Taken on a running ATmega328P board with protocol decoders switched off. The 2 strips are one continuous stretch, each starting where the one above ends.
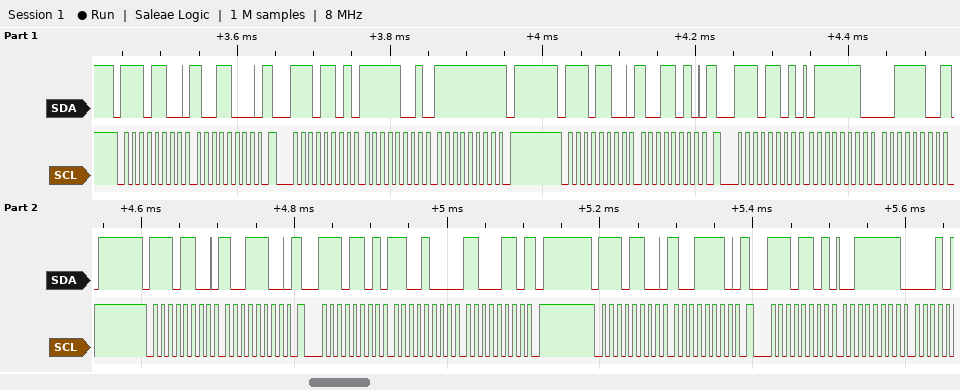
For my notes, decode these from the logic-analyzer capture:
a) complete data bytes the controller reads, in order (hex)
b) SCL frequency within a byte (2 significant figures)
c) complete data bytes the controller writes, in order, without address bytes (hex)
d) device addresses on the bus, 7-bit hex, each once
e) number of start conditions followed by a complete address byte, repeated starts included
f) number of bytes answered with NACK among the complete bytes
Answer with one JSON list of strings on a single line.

["F9 FF 7E 3C C8 C6 3F", "100 kHz", "98 9A 9C 9E", "0x76", "8", "3"]
